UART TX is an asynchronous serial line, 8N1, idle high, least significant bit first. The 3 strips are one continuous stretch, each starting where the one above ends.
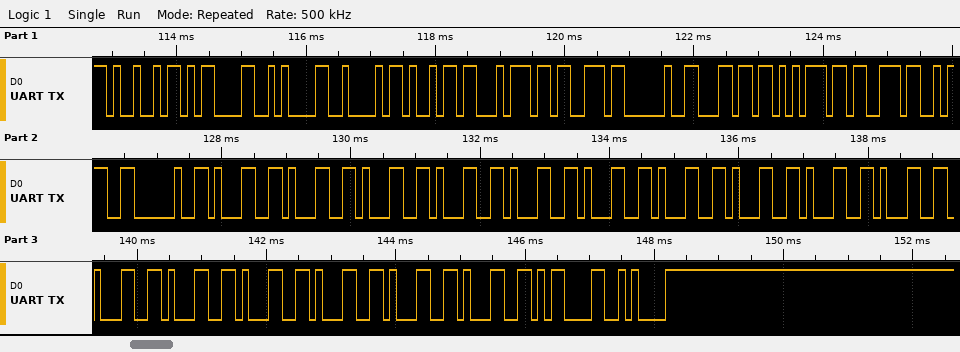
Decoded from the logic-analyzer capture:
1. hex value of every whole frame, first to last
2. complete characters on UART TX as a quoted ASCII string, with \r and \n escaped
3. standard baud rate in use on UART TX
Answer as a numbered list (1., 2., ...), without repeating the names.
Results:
1. 0x49 0x0D 0x0A 0x42 0x69 0x74 0x73 0x20 0x6C 0x75 0x73 0x3A 0x20 0x31 0x31 0x31 0x31 0x31 0x31 0x31 0x31 0x31 0x31 0x31 0x31 0x31 0x31 0x31 0x31 0x0D 0x0A
2. "I\r\nBits lus: 1111111111111111\r\n"
3. 9600 baud
